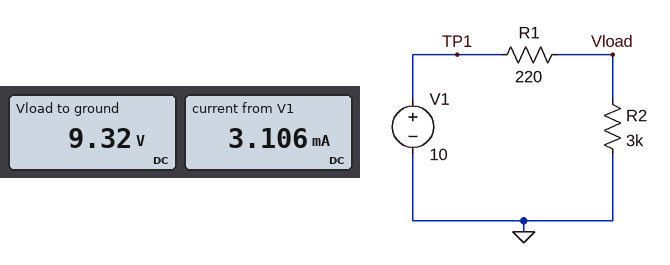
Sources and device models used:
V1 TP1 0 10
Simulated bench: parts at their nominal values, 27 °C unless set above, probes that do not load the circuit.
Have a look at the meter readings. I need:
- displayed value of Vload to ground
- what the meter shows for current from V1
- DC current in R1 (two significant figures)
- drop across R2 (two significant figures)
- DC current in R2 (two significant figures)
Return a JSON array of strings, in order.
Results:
["9.32 V", "3.106 mA", "3.1 mA", "9.3 V", "3.1 mA"]
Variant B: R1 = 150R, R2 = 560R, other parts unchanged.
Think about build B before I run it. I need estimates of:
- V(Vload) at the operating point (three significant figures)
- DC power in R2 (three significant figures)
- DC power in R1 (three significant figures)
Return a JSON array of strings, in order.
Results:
["7.89 V", "111 mW", "29.8 mW"]
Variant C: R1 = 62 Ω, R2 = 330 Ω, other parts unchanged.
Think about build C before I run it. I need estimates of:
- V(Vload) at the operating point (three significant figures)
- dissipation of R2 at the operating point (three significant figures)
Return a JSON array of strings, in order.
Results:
["8.42 V", "215 mW"]
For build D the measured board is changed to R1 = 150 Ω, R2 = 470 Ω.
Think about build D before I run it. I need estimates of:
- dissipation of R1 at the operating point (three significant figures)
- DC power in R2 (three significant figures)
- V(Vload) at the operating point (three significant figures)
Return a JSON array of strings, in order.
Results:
["39.0 mW", "122 mW", "7.58 V"]
